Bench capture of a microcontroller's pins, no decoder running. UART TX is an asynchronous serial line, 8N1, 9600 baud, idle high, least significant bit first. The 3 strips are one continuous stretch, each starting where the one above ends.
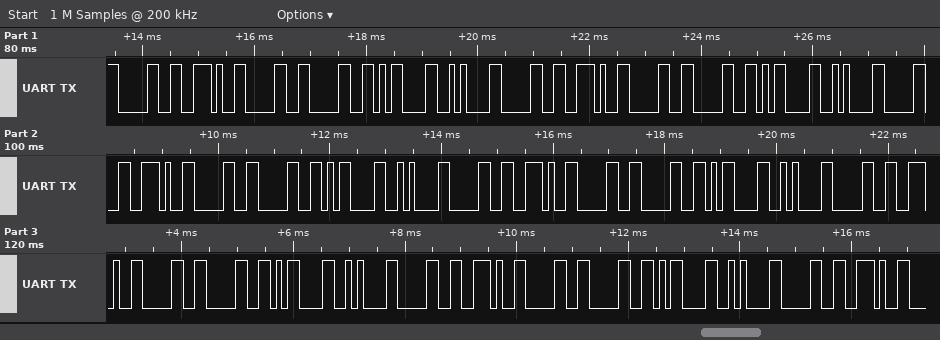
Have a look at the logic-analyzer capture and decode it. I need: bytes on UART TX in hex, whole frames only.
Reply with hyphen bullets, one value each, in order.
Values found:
- 30 2E 30 30 0D 0A 30 2E 30 30 0D 0A 30 2E 30 30 0D 0A 30 2E 30 30 0D 0A 30 2E 30 30 0D 0A 30 2E 30 30 0D 0A 30 2E
